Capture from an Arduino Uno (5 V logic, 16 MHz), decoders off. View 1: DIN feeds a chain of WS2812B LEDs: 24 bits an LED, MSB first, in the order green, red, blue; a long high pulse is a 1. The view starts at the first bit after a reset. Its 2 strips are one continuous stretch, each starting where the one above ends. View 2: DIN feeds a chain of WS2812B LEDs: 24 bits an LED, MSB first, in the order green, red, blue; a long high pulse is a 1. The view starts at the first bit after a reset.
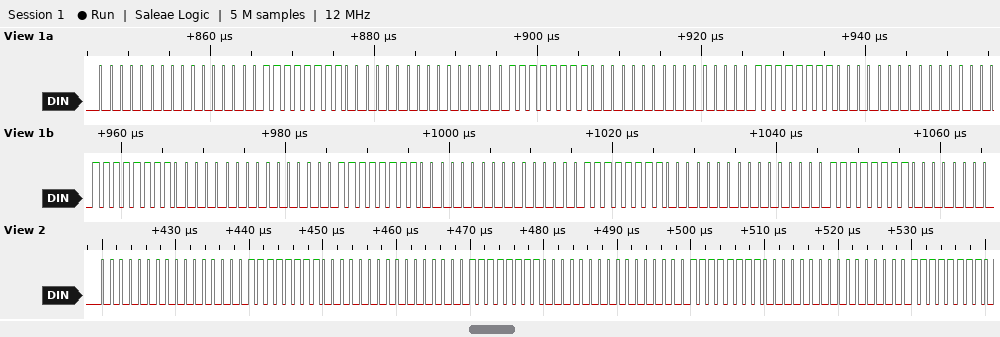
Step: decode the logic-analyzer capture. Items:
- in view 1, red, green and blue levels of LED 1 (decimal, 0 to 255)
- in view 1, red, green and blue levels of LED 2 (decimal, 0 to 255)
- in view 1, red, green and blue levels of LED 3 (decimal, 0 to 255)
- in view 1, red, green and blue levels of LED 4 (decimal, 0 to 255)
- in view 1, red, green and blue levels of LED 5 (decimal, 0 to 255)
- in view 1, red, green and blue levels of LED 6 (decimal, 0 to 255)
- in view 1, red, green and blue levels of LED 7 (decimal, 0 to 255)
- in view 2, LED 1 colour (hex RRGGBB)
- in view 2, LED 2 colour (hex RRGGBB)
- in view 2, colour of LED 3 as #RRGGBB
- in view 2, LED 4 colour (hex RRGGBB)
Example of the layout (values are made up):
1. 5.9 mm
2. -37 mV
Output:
1. 0, 0, 255
2. 0, 0, 255
3. 0, 0, 255
4. 0, 0, 255
5. 0, 0, 255
6. 0, 0, 255
7. 0, 0, 255
8. #0000FF
9. #0000FF
10. #0000FF
11. #0000FF
